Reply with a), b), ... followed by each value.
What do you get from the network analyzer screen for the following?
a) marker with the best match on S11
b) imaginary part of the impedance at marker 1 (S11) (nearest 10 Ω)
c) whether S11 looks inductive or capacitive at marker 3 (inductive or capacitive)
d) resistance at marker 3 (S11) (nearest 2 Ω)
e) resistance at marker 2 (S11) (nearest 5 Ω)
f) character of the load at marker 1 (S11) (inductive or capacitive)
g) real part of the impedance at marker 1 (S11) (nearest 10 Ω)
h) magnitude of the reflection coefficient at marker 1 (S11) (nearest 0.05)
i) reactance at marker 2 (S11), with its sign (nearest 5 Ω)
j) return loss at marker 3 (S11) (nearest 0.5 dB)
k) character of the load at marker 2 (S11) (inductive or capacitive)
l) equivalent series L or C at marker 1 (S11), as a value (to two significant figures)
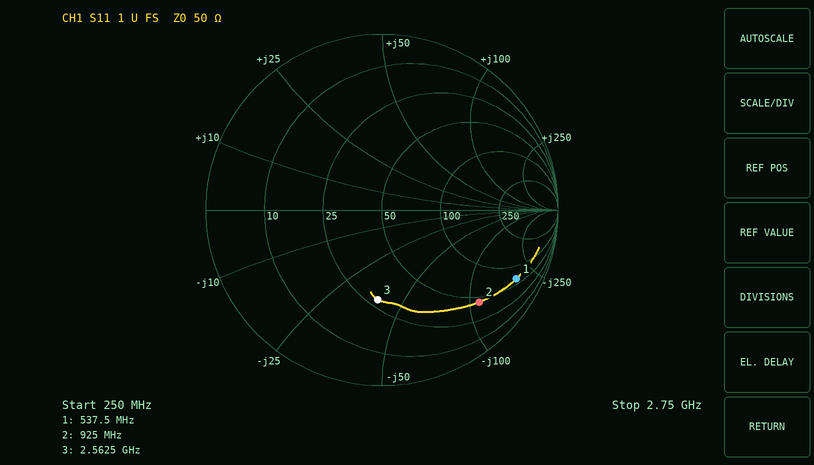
a) marker 3
b) -190 Ω
c) capacitive
d) 28 Ω
e) 45 Ω
f) capacitive
g) 60 Ω
h) 0.85
i) -110 Ω
j) 6.0 dB
k) capacitive
l) 1.6 pF
